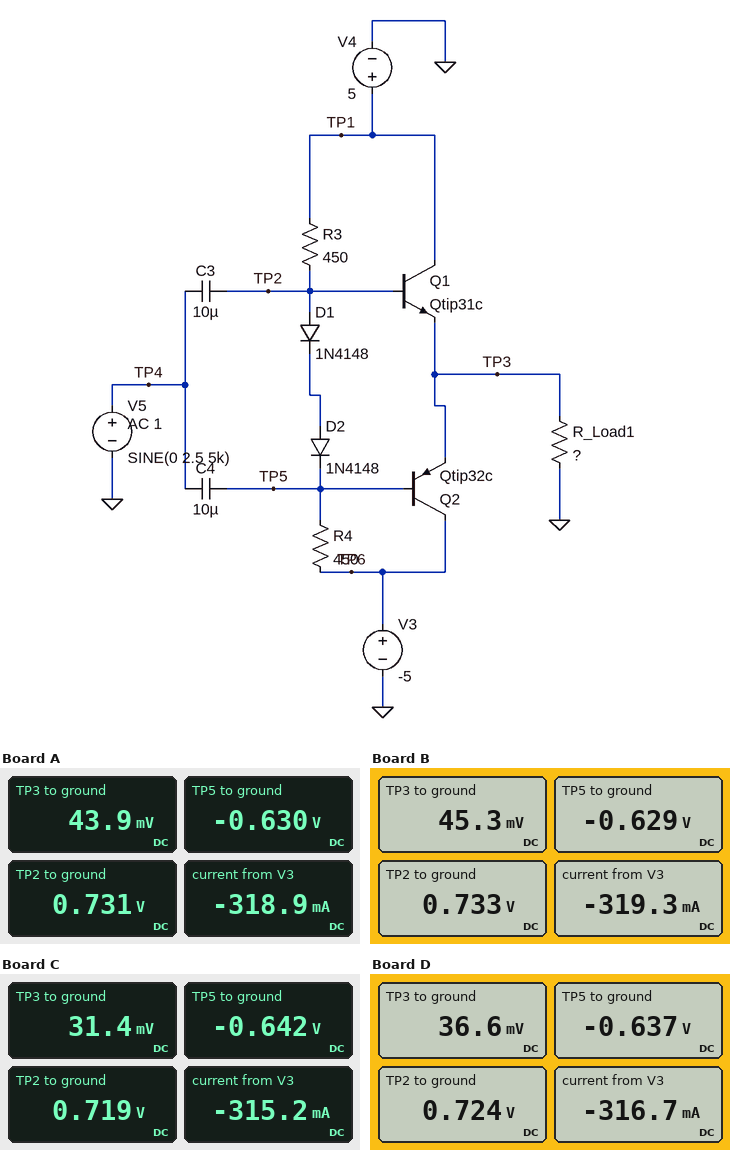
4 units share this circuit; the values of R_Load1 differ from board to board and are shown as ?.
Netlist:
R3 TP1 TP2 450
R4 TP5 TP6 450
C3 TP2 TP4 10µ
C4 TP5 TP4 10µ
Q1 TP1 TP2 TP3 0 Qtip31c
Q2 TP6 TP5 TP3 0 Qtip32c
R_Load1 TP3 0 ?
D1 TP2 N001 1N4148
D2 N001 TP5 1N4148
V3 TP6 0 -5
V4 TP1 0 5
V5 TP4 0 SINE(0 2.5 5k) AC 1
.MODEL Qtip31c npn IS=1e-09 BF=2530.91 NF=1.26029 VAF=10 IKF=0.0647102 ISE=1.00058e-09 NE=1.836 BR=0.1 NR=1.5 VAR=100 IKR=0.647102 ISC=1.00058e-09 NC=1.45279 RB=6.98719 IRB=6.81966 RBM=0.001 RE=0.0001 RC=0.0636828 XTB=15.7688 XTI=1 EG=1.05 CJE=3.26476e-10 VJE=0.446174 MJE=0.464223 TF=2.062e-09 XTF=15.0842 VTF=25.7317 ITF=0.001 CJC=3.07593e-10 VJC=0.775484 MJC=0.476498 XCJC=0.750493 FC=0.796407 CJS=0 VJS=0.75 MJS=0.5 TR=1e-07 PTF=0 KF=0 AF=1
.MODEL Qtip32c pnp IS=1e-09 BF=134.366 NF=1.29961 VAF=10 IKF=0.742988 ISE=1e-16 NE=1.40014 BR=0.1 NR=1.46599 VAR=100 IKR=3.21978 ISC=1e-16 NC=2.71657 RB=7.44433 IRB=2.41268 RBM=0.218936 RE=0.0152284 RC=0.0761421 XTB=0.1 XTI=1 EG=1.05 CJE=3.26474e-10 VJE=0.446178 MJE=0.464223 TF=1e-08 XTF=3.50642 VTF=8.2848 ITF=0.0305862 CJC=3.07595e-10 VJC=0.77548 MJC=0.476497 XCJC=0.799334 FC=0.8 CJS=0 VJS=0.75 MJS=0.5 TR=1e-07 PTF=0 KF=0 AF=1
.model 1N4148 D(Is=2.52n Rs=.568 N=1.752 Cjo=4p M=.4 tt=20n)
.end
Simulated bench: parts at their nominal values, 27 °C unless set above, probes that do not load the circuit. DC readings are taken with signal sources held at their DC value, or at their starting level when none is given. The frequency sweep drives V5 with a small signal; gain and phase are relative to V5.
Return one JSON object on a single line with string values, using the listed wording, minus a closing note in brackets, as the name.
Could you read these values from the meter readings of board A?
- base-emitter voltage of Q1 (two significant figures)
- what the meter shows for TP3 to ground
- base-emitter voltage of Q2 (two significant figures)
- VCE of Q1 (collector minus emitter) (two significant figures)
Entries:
{"base-emitter voltage of Q1": "690 mV", "what the meter shows for TP3 to ground": "43.9 mV", "base-emitter voltage of Q2": "-670 mV", "VCE of Q1 (collector minus emitter)": "5.0 V"}
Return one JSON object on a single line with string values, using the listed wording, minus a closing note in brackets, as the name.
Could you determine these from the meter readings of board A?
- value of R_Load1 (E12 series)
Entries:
{"value of R_Load1": "18 Ω"}
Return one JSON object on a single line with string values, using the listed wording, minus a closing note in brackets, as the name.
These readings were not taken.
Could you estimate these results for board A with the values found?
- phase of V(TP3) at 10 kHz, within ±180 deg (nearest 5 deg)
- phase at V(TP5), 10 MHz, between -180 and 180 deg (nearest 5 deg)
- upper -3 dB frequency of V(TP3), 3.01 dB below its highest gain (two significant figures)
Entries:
{"phase of V(TP3) at 10 kHz, within ±180 deg": "0 deg", "phase at V(TP5), 10 MHz, between -180 and 180 deg": "0 deg", "upper -3 dB frequency of V(TP3), 3.01 dB below its highest gain": "130 MHz"}
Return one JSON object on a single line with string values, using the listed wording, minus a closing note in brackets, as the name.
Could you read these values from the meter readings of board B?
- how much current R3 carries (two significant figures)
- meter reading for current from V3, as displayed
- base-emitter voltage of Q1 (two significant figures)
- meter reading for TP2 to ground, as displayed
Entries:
{"how much current R3 carries": "9.5 mA", "meter reading for current from V3, as displayed": "-319.3 mA", "base-emitter voltage of Q1": "690 mV", "meter reading for TP2 to ground, as displayed": "0.733 V"}
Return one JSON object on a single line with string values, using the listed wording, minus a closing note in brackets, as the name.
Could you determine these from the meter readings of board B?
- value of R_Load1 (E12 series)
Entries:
{"value of R_Load1": "27 Ω"}
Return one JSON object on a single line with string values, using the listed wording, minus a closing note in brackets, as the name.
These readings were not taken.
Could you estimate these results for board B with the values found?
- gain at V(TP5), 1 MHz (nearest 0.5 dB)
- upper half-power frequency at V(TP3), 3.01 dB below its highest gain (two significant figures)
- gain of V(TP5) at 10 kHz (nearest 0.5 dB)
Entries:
{"gain at V(TP5), 1 MHz": "0 dB", "upper half-power frequency at V(TP3), 3.01 dB below its highest gain": "160 MHz", "gain of V(TP5) at 10 kHz": "0 dB"}
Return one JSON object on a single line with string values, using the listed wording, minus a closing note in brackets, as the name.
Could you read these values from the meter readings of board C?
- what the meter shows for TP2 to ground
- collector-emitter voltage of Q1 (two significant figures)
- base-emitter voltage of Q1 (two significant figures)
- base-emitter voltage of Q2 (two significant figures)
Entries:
{"what the meter shows for TP2 to ground": "0.719 V", "collector-emitter voltage of Q1": "5.0 V", "base-emitter voltage of Q1": "690 mV", "base-emitter voltage of Q2": "-670 mV"}
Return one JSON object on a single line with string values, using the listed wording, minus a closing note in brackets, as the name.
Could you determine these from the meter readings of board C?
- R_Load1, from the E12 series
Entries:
{"R_Load1, from the E12 series": "3.3 Ω"}
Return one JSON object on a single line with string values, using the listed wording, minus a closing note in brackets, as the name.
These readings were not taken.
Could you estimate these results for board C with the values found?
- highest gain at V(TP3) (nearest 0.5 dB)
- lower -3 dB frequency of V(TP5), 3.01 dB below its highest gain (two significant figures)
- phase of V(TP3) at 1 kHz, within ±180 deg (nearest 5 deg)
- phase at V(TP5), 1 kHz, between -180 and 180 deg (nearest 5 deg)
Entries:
{"highest gain at V(TP3)": "-0.5 dB", "lower -3 dB frequency of V(TP5), 3.01 dB below its highest gain": "57 Hz", "phase of V(TP3) at 1 kHz, within ±180 deg": "5 deg", "phase at V(TP5), 1 kHz, between -180 and 180 deg": "5 deg"}
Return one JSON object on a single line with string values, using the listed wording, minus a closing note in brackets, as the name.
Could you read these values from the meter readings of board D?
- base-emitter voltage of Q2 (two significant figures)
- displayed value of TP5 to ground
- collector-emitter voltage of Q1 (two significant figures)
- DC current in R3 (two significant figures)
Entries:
{"base-emitter voltage of Q2": "-670 mV", "displayed value of TP5 to ground": "-0.637 V", "collector-emitter voltage of Q1": "5.0 V", "DC current in R3": "9.5 mA"}
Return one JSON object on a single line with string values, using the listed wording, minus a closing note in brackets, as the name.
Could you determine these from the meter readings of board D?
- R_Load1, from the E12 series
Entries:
{"R_Load1, from the E12 series": "5.6 Ω"}
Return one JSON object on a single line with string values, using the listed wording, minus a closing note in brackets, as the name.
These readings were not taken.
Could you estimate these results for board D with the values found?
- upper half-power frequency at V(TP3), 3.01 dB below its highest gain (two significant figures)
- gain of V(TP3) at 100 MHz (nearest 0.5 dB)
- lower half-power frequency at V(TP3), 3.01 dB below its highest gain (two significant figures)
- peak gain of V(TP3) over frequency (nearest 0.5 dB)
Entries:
{"upper half-power frequency at V(TP3), 3.01 dB below its highest gain": "5.2 MHz", "gain of V(TP3) at 100 MHz": "-5.0 dB", "lower half-power frequency at V(TP3), 3.01 dB below its highest gain": "49 Hz", "peak gain of V(TP3) over frequency": "0 dB"}
